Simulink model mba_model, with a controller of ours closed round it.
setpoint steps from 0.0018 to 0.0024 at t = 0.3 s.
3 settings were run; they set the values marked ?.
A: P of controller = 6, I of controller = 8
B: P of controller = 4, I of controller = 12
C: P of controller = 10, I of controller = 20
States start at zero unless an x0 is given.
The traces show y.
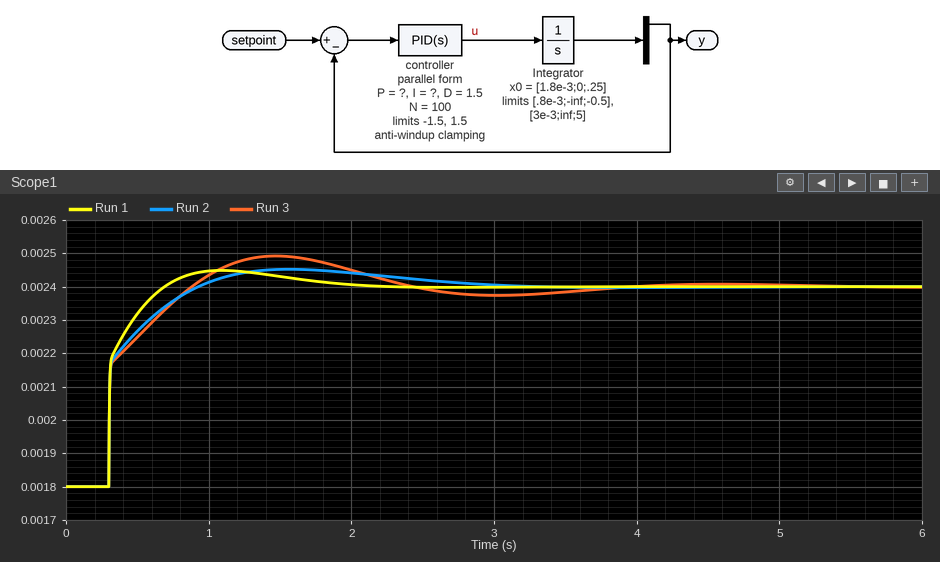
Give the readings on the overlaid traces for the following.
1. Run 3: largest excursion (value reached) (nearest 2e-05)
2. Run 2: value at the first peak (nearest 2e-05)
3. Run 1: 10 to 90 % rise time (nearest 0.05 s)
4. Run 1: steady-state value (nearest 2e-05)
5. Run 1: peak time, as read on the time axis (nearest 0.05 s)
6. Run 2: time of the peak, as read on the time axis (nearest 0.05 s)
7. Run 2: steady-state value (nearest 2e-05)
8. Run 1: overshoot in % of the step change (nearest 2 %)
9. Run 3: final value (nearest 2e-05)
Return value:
0.00250
0.00246
0.25 s
0.00240
1.10 s
1.55 s
0.00240
8 %
0.00240
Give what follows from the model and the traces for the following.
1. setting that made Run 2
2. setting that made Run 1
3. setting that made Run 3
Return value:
A
C
B
